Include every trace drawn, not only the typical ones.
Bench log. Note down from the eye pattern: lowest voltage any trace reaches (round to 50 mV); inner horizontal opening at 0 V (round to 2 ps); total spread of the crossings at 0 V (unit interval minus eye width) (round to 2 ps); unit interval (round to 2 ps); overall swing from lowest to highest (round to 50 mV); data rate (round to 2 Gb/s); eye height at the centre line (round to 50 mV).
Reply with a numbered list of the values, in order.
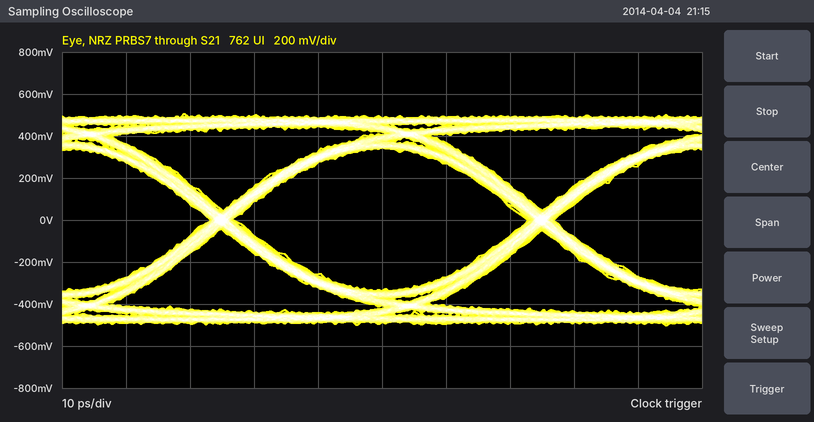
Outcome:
1. -500 mV
2. 46 ps
3. 4 ps
4. 50 ps
5. 1.00 V
6. 20 Gb/s
7. 700 mV
